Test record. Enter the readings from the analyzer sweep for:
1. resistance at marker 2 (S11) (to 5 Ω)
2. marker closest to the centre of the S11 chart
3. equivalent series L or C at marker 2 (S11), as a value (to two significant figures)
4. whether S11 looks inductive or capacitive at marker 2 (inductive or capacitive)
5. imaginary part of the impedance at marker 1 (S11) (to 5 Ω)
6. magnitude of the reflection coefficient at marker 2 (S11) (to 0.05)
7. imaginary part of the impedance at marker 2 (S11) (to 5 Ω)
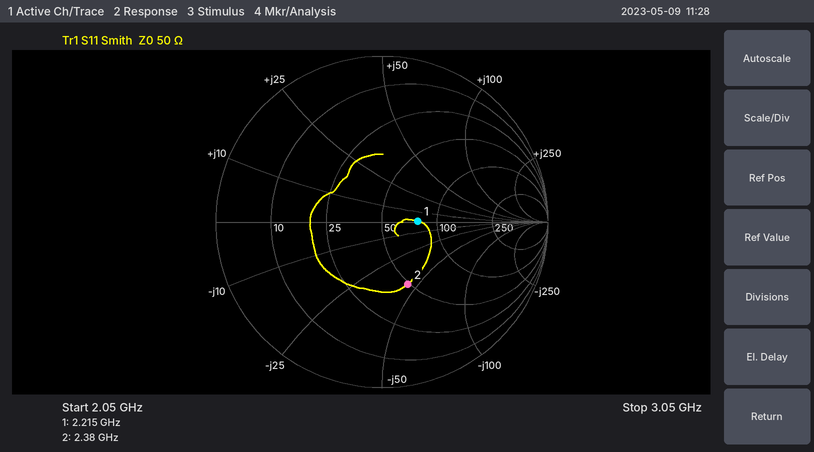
50 Ω
marker 1
1.5 pF
capacitive
0 Ω
0.40
-45 Ω
